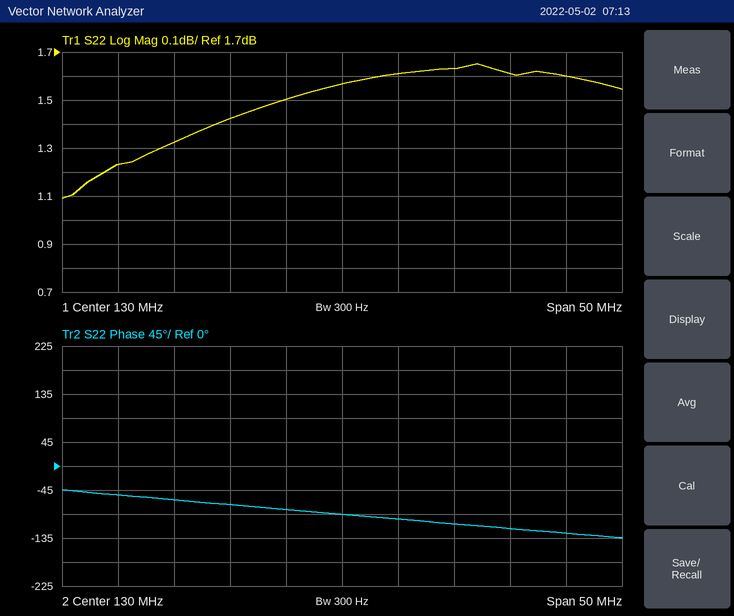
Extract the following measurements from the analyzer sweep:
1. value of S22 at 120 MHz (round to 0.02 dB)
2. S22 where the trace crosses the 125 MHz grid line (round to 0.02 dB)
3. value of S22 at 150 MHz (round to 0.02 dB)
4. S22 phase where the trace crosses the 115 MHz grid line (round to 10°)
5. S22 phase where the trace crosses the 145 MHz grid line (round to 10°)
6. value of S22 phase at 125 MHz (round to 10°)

1.42 dB
1.50 dB
1.60 dB
-60°
-120°
-80°
